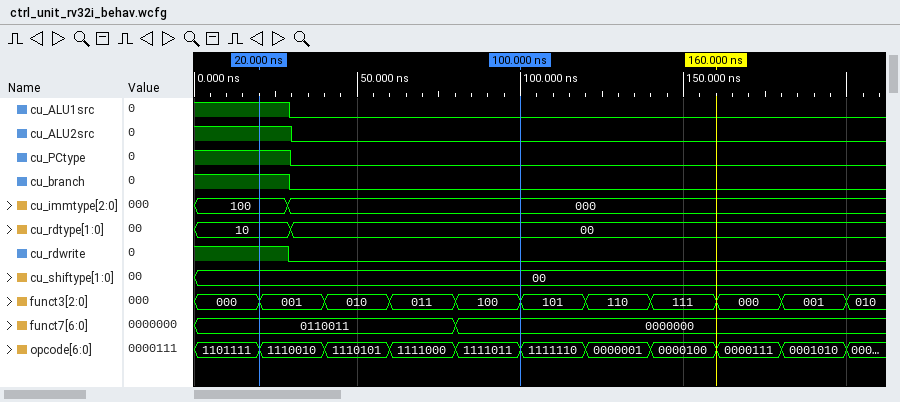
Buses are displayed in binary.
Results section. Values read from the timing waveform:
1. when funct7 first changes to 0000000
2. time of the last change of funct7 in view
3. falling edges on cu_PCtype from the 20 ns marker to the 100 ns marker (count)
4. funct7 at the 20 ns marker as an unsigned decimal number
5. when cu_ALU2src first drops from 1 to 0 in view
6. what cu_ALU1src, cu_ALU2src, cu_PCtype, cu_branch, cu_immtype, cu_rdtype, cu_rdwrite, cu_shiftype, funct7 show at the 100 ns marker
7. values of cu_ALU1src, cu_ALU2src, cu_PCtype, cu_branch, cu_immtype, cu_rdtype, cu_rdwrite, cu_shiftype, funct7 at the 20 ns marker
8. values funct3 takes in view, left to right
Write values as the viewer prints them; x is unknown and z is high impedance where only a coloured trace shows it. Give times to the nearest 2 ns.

80 ns
80 ns
1
51
30 ns
cu_ALU1src=0, cu_ALU2src=0, cu_PCtype=0, cu_branch=0, cu_immtype=000, cu_rdtype=00, cu_rdwrite=0, cu_shiftype=00, funct7=0000000
cu_ALU1src=1, cu_ALU2src=1, cu_PCtype=1, cu_branch=1, cu_immtype=100, cu_rdtype=10, cu_rdwrite=1, cu_shiftype=00, funct7=0110011
000, 001, 010, 011, 100, 101, 110, 111, 000, 001, 010
